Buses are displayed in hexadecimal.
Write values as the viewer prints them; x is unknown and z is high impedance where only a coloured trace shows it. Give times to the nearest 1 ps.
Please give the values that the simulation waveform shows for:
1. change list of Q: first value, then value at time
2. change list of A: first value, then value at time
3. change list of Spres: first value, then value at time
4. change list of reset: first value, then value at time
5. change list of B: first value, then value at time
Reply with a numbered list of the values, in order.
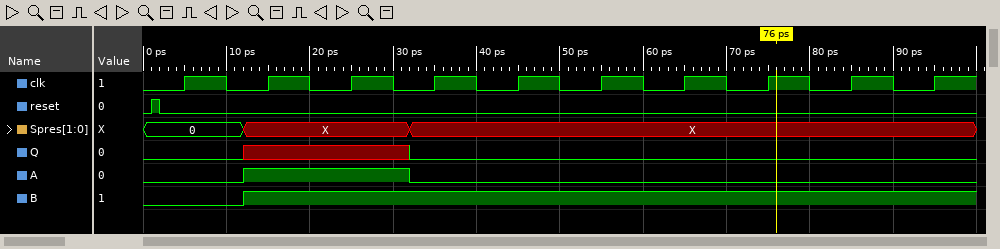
1. 0, x at 12 ps, 0 at 32 ps
2. 0, 1 at 12 ps, 0 at 32 ps
3. 0, X at 12 ps, X at 32 ps
4. 0, 1 at 1 ps, 0 at 2 ps
5. 0, 1 at 12 ps
